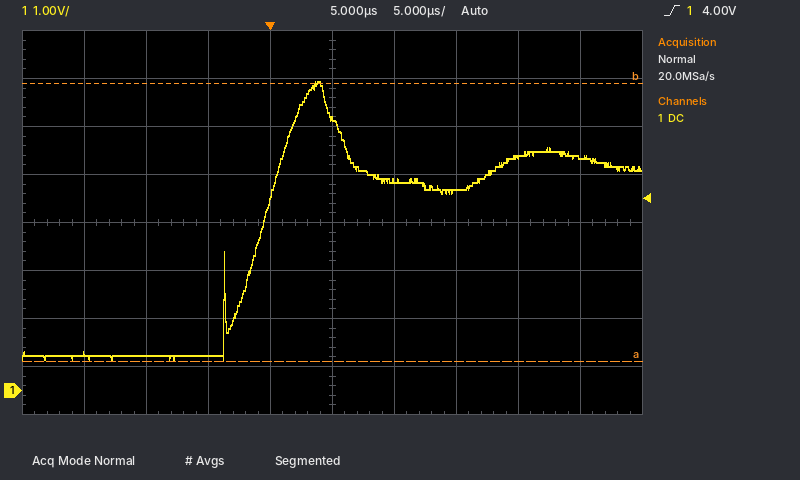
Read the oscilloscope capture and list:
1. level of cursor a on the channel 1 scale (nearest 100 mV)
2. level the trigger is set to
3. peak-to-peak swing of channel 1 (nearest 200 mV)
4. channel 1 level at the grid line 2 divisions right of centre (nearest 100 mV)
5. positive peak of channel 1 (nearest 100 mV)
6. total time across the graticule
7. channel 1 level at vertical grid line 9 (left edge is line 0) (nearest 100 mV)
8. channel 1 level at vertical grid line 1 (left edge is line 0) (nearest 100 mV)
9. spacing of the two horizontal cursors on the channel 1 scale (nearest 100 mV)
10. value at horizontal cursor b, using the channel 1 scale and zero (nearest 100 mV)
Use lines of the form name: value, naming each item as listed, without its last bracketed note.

level of cursor a on the channel 1 scale: 600 mV
level the trigger is set to: 4.00 V
peak-to-peak swing of channel 1: 5.8 V
channel 1 level at the grid line 2 divisions right of centre: 4.2 V
positive peak of channel 1: 6.4 V
total time across the graticule: 50 µs
channel 1 level at vertical grid line 9 (left edge is line 0): 4.9 V
channel 1 level at vertical grid line 1 (left edge is line 0): 800 mV
spacing of the two horizontal cursors on the channel 1 scale: 5.8 V
value at horizontal cursor b, using the channel 1 scale and zero: 6.4 V
